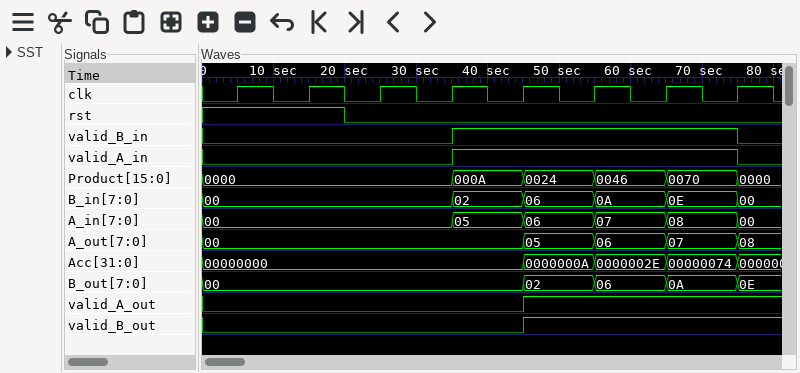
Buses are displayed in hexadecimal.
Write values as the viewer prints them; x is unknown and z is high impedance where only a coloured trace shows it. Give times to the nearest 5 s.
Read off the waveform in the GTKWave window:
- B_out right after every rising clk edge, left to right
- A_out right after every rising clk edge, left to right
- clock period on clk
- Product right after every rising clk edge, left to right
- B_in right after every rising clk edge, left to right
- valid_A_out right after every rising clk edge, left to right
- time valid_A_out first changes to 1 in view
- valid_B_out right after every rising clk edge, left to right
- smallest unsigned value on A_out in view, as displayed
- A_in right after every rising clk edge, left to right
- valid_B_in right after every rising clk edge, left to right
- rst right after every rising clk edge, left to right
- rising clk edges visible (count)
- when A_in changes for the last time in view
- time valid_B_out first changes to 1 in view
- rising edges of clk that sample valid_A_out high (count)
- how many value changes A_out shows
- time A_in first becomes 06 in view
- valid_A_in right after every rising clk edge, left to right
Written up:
00, 00, 00, 00, 02, 06, 0A, 0E
00, 00, 00, 00, 05, 06, 07, 08
10 s
0000, 0000, 0000, 000A, 0024, 0046, 0070, 0000
00, 00, 00, 02, 06, 0A, 0E, 00
0 0 0 0 1 1 1 1
45 s
0 0 0 0 1 1 1 1
00
00, 00, 00, 05, 06, 07, 08, 00
0 0 0 1 1 1 1 0
1 1 0 0 0 0 0 0
8
75 s
45 s
3
4
45 s
0 0 0 1 1 1 1 0
